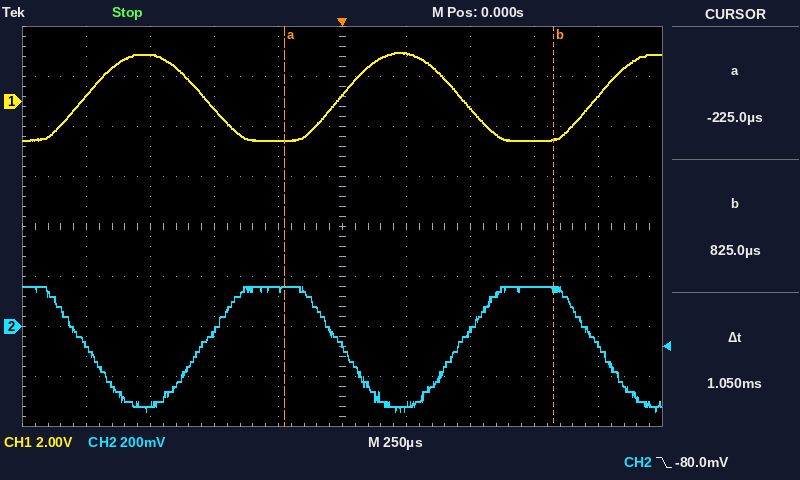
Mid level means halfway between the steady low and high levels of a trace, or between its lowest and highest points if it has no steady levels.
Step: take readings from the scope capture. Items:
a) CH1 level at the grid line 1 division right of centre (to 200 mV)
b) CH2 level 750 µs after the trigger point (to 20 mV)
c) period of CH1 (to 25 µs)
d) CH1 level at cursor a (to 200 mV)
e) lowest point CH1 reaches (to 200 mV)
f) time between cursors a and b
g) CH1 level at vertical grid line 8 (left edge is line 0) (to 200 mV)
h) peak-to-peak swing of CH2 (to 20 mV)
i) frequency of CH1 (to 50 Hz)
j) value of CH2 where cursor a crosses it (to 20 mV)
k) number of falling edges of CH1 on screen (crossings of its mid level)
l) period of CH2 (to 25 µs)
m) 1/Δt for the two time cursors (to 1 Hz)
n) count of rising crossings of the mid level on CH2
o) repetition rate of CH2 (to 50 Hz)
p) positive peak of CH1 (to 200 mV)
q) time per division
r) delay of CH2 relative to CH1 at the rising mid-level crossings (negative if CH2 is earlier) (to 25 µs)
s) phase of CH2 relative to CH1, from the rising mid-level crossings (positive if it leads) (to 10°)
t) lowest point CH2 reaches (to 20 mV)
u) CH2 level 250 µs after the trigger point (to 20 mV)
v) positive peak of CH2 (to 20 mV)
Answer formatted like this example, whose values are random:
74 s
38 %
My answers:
2.0 V
160 mV
1.000 ms
-1.6 V
-1.6 V
1.05 ms
-1.6 V
500 mV
1.00 kHz
160 mV
2
1.000 ms
952 Hz
2
1.00 kHz
2.0 V
250 µs
+450 µs
-160°
-340 mV
-320 mV
160 mV
